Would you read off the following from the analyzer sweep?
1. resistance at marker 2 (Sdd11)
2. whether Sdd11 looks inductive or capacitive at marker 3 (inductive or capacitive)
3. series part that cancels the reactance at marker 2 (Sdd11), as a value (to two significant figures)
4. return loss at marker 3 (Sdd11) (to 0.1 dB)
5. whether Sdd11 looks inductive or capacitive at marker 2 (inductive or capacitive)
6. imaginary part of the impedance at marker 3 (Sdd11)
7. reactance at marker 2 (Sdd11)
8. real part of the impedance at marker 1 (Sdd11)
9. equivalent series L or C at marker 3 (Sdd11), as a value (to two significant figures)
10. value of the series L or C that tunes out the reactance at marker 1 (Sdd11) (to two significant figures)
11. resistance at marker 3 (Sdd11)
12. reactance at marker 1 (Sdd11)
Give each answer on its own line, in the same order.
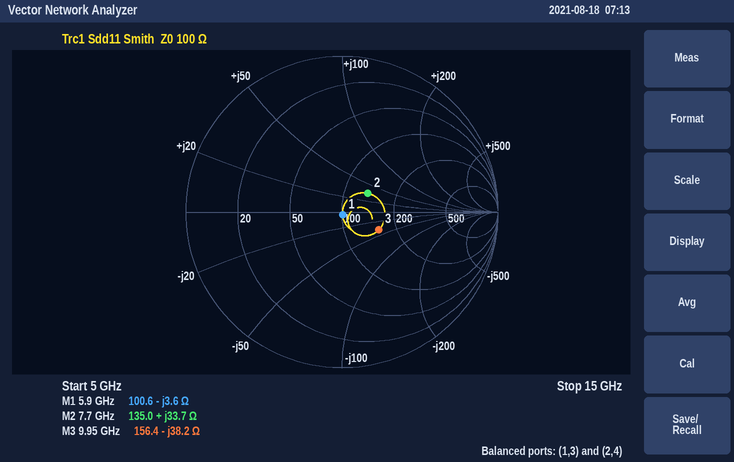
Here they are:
135.0 Ω
capacitive
610 fF
11.6 dB
inductive
-38.2 Ω
+33.7 Ω
100.6 Ω
420 fF
97 pH
156.4 Ω
-3.6 Ω
